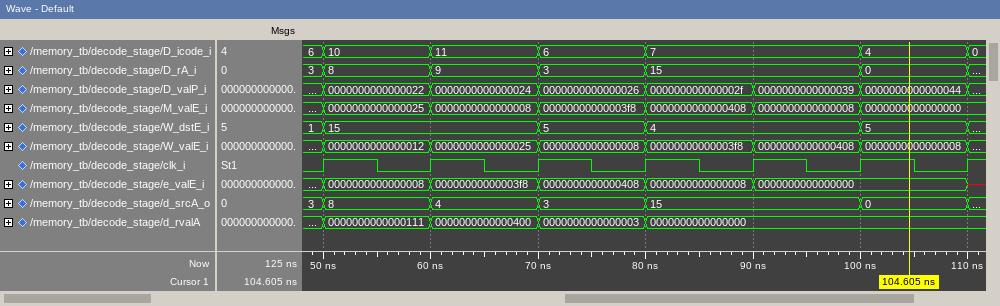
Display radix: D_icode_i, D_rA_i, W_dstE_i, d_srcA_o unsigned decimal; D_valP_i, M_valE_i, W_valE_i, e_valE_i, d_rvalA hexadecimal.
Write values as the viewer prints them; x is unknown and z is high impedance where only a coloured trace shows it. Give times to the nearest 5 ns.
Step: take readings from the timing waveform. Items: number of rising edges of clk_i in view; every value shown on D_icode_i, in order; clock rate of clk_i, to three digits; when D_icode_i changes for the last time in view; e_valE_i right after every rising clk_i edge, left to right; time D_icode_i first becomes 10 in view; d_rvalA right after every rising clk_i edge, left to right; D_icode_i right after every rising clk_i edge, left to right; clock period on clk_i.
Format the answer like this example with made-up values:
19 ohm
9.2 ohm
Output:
7
6, 10, 11, 6, 7, 4, 0
100 MHz
110 ns
0000000000000008, 00000000000003f8, 0000000000000408, 0000000000000008, 0000000000000000, 0000000000000000, x
50 ns
0000000000000111, 0000000000000400, 0000000000000003, 0000000000000000, 0000000000000000, 0000000000000000, 0000000000000000
10, 11, 6, 7, 7, 4, 0
10 ns
